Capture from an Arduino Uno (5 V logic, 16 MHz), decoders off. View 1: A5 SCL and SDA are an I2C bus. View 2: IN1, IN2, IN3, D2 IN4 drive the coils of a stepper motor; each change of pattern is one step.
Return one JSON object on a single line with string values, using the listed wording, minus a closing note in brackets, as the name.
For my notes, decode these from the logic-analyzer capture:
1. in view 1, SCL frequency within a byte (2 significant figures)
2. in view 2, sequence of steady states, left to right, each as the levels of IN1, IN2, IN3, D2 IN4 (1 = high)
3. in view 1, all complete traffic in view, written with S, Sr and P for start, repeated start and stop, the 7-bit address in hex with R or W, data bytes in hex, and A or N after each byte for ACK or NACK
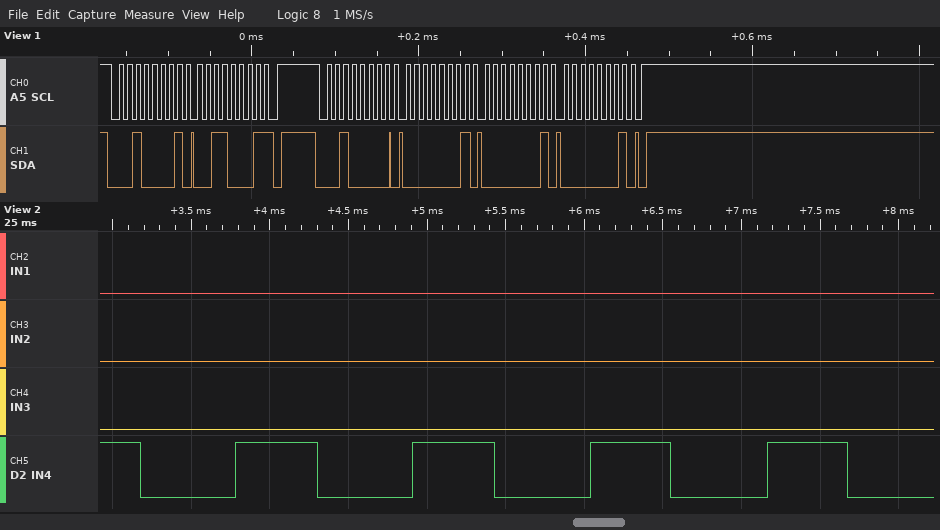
{"in view 1, SCL frequency within a byte": "100 kHz", "in view 2, sequence of steady states, left to right, each as the levels of IN1, IN2, IN3, D2 IN4": "0001 0000 0001 0000 0001 0000 0001 0000 0001 0000", "in view 1, all complete traffic in view, written with S, Sr and P for start, repeated start and stop, the 7-bit address in hex with R or W, data bytes in hex, and A or N after each byte for ACK or NACK": "S 10R A 31 N P S 10W A 01 A 01 A 01 A P"}
